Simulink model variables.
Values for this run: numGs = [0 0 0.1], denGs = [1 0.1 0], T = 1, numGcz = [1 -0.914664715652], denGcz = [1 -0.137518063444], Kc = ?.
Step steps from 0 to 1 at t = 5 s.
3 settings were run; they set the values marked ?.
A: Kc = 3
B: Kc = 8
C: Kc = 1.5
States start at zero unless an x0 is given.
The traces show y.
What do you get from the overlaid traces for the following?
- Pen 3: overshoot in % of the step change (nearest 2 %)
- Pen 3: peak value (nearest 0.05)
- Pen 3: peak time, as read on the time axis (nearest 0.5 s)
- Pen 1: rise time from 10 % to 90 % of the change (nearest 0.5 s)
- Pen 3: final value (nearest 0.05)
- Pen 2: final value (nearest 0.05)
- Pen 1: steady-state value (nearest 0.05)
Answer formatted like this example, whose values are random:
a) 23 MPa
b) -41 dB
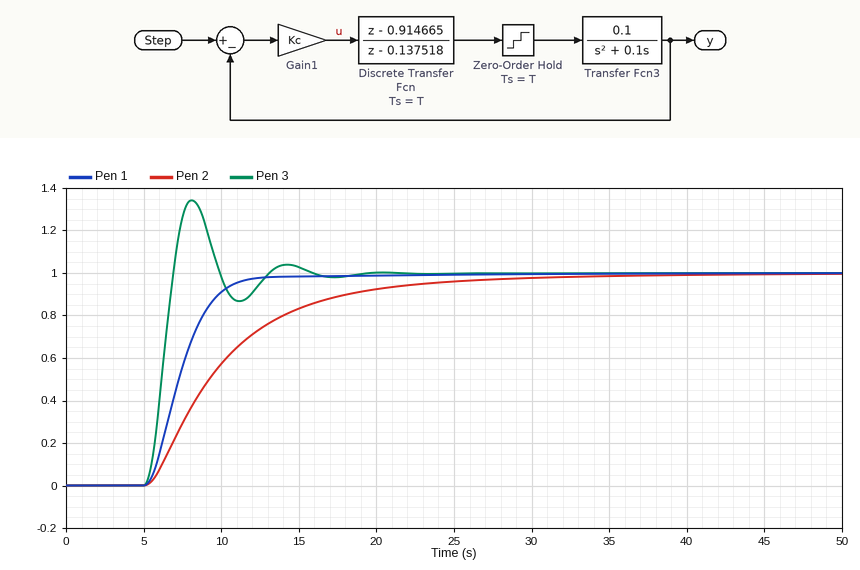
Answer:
a) 34 %
b) 1.35
c) 8.0 s
d) 4.0 s
e) 1.00
f) 1.00
g) 1.00
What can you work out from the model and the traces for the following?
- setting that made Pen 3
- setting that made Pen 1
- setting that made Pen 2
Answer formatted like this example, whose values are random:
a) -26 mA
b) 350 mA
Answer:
a) B
b) A
c) C
